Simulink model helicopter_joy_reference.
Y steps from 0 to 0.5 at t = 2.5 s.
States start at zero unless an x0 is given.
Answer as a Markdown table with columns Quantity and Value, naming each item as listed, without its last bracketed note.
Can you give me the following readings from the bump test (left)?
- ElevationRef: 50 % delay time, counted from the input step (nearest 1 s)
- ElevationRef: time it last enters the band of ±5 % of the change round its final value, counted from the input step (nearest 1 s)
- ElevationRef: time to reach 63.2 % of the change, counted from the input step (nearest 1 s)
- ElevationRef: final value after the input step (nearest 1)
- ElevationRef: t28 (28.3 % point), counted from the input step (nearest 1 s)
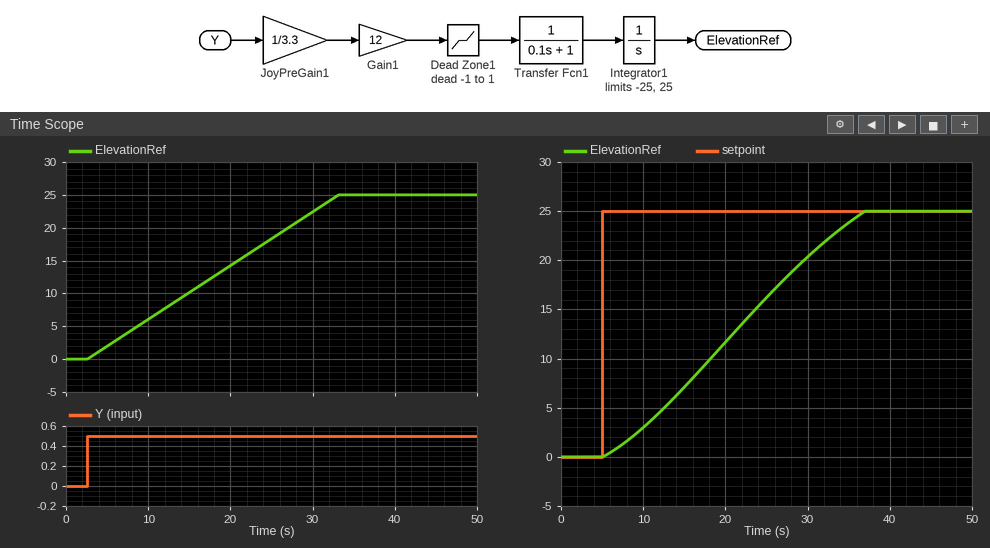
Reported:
| Quantity | Value |
|---|---|
| ElevationRef: 50 % delay time, counted from the input step | 15 s |
| ElevationRef: time it last enters the band of ±5 % of the change round its final value, counted from the input step | 29 s |
| ElevationRef: time to reach 63.2 % of the change, counted from the input step | 19 s |
| ElevationRef: final value after the input step | 25 |
| ElevationRef: t28 (28.3 % point), counted from the input step | 9 s |
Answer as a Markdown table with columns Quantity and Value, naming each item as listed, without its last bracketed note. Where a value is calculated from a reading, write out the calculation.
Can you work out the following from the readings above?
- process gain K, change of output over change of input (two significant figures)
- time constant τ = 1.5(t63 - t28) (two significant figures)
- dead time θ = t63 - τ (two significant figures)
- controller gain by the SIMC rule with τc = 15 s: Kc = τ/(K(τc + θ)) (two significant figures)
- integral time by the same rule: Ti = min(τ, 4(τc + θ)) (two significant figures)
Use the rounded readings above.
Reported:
| Quantity | Value |
|---|---|
| process gain K, change of output over change of input | (25 - 0) / 0.5 = 50 |
| time constant τ = 1.5(t63 - t28) | 1.5 × (19 - 9) = 15 s |
| dead time θ = t63 - τ | 19 - 15 = 4.0 s |
| controller gain by the SIMC rule with τc = 15 s: Kc = τ/(K(τc + θ)) | 15 / (50 × (15 + 4)) = 0.016 |
| integral time by the same rule: Ti = min(τ, 4(τc + θ)) | min(15, 4 × (15 + 4)) = 15 s |
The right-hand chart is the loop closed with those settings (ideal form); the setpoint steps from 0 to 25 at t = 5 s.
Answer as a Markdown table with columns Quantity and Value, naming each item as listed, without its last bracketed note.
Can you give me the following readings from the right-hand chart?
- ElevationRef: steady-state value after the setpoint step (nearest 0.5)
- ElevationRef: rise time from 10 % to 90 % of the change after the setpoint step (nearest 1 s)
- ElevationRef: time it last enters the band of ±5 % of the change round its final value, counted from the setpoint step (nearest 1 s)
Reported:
| Quantity | Value |
|---|---|
| ElevationRef: steady-state value after the setpoint step | 25.0 |
| ElevationRef: rise time from 10 % to 90 % of the change after the setpoint step | 24 s |
| ElevationRef: time it last enters the band of ±5 % of the change round its final value, counted from the setpoint step | 30 s |
